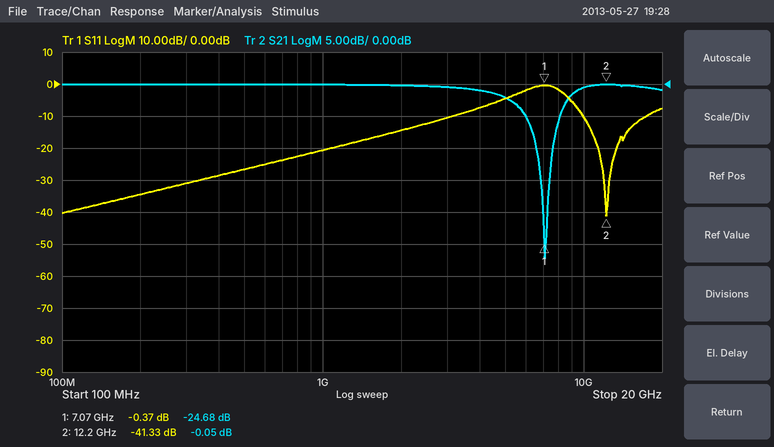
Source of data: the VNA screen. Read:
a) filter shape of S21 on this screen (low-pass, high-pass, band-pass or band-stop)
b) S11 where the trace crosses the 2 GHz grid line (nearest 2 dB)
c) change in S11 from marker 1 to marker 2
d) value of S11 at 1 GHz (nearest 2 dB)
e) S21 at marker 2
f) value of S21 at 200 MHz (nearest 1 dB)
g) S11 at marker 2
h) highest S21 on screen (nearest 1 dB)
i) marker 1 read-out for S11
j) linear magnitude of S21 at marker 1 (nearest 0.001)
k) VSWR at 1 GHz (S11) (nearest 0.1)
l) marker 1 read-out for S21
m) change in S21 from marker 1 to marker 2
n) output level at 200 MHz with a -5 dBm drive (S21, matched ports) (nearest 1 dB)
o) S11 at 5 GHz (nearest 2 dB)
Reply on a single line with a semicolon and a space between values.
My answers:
band-stop; -14 dB; -40.96 dB; -20 dB; -0.05 dB; 0 dB; -41.33 dB; 0 dB; -0.37 dB; 0.058; 1.2; -24.68 dB; 24.63 dB; -5 dBm; -4 dB
